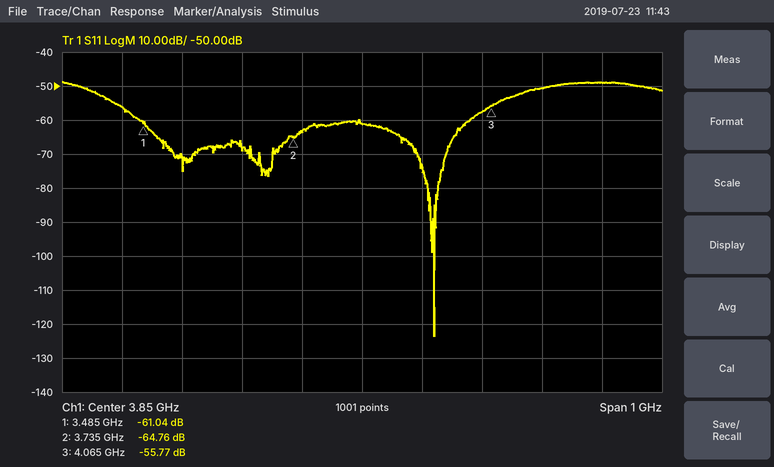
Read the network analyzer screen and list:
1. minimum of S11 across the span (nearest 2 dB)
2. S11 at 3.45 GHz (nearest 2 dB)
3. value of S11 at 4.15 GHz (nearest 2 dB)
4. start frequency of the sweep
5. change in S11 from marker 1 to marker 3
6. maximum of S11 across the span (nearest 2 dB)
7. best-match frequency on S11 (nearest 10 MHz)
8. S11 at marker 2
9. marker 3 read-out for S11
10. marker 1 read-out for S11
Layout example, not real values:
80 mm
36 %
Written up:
-124 dB
-56 dB
-50 dB
3.35 GHz
5.27 dB
-48 dB
3.97 GHz
-64.76 dB
-55.77 dB
-61.04 dB
